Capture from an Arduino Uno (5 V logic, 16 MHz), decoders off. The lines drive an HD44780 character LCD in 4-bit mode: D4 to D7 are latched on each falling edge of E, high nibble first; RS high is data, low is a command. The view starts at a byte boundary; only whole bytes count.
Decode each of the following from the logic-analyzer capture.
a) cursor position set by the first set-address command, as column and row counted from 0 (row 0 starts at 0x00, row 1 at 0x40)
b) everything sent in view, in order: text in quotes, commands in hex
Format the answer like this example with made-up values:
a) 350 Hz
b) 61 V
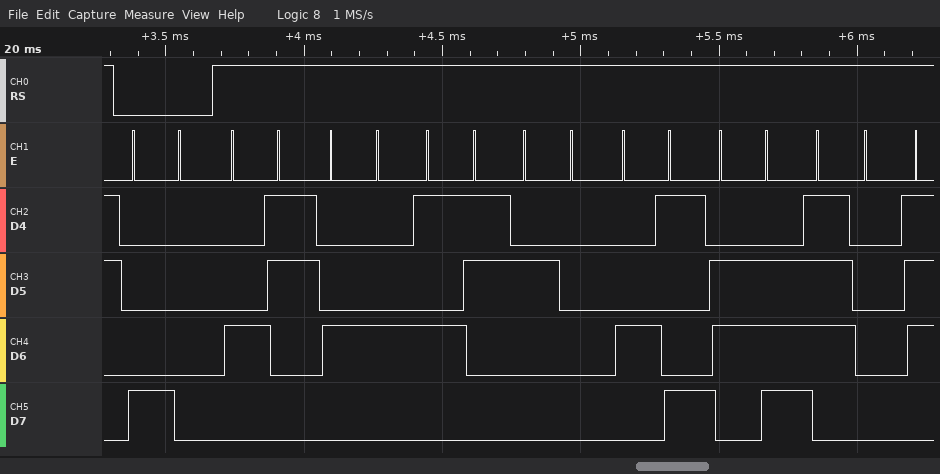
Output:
a) column 0, row 0
b) 0x80 "CDS Inp"
